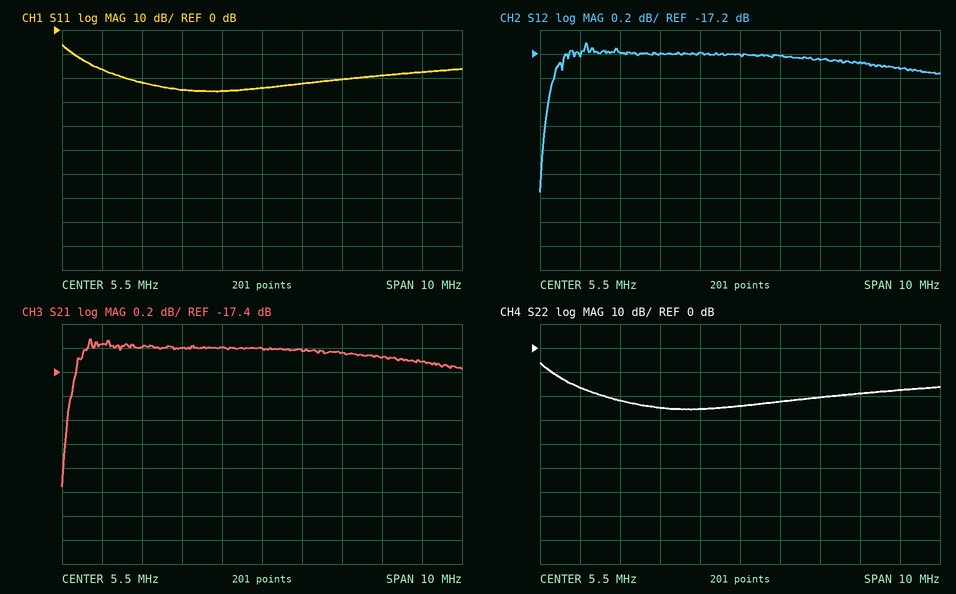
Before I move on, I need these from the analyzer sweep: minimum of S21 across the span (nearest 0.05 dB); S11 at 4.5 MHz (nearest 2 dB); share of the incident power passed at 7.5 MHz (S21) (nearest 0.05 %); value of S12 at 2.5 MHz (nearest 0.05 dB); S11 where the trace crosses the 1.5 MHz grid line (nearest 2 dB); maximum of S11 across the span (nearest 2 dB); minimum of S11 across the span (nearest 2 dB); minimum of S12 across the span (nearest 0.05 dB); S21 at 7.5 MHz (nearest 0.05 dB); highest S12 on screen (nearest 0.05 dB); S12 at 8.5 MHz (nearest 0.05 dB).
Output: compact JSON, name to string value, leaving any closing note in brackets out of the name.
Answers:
{"minimum of S21 across the span": "-18.35 dB", "S11 at 4.5 MHz": "-26 dB", "share of the incident power passed at 7.5 MHz (S21)": "1.90 %", "value of S12 at 2.5 MHz": "-17.20 dB", "S11 where the trace crosses the 1.5 MHz grid line": "-16 dB", "maximum of S11 across the span": "-6 dB", "minimum of S11 across the span": "-26 dB", "minimum of S12 across the span": "-18.35 dB", "S21 at 7.5 MHz": "-17.25 dB", "highest S12 on screen": "-17.10 dB", "S12 at 8.5 MHz": "-17.25 dB"}
